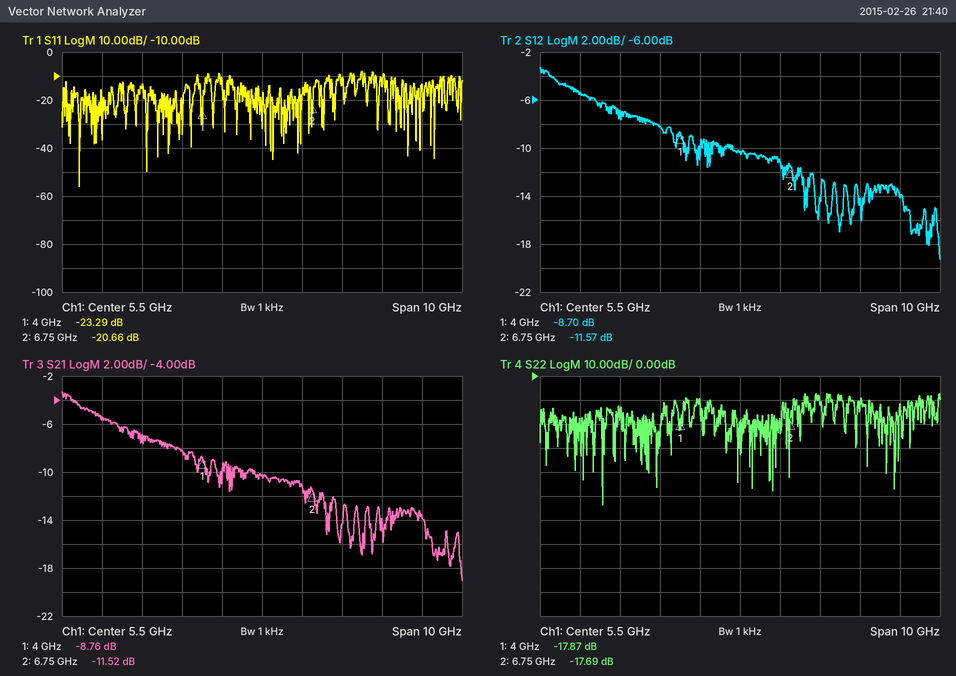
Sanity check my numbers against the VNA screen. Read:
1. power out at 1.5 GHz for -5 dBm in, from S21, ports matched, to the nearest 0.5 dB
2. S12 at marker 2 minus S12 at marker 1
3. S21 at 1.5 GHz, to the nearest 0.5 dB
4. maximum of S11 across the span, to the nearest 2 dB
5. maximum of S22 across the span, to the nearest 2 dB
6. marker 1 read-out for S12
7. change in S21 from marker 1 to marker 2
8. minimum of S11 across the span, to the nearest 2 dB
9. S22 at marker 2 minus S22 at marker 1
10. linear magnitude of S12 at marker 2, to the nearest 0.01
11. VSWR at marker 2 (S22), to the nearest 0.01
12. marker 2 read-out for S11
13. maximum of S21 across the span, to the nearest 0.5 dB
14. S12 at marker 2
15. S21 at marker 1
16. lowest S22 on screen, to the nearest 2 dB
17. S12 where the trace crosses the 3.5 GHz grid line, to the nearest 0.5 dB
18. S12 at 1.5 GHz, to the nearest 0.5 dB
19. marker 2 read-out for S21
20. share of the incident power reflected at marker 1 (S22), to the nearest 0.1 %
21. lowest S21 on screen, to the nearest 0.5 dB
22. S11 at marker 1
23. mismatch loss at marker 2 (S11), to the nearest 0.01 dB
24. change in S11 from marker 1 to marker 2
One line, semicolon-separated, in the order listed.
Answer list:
-10.5 dBm; -2.87 dB; -5.5 dB; -8 dB; -8 dB; -8.70 dB; -2.76 dB; -56 dB; 0.18 dB; 0.26; 1.30; -20.66 dB; -3.5 dB; -11.57 dB; -8.76 dB; -54 dB; -8.0 dB; -5.5 dB; -11.52 dB; 1.6 %; -19.0 dB; -23.29 dB; 0.04 dB; 2.63 dB
